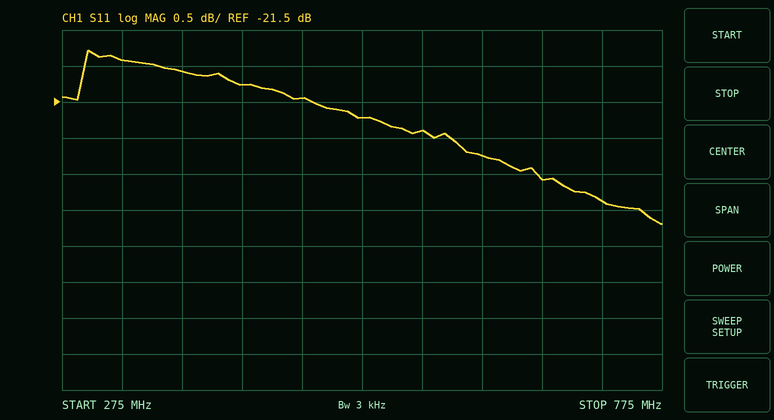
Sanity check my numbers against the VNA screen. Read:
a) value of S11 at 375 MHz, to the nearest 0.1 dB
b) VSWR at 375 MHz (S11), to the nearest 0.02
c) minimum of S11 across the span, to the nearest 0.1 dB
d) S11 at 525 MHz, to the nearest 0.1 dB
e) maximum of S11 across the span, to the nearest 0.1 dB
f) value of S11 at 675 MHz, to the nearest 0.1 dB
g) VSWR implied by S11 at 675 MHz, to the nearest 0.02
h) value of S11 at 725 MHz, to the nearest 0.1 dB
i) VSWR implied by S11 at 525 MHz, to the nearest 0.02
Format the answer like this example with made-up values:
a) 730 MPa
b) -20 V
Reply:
a) -21.1 dB
b) 1.20
c) -23.2 dB
d) -21.7 dB
e) -20.8 dB
f) -22.6 dB
g) 1.16
h) -22.9 dB
i) 1.18
